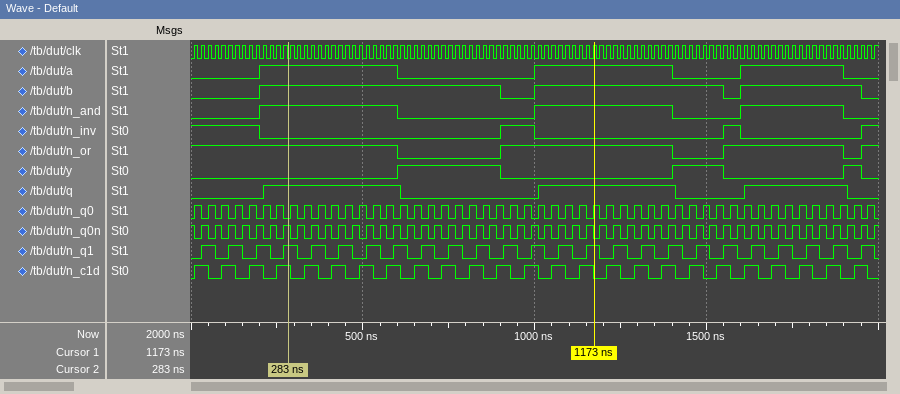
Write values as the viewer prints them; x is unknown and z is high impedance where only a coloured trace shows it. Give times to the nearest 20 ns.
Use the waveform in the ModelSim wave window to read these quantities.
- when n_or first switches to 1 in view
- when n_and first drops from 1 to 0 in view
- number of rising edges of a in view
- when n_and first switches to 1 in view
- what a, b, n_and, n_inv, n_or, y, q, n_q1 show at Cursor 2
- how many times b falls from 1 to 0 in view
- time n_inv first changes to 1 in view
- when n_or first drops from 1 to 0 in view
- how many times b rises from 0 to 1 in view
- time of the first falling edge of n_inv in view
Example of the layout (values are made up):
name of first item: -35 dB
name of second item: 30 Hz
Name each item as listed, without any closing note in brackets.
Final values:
when n_or first switches to 1 in view: 900 ns
when n_and first drops from 1 to 0 in view: 600 ns
number of rising edges of a in view: 3
when n_and first switches to 1 in view: 200 ns
what a, b, n_and, n_inv, n_or, y, q, n_q1 show at Cursor 2: a=1, b=1, n_and=1, n_inv=0, n_or=1, y=0, q=1, n_q1=1
how many times b falls from 1 to 0 in view: 3
time n_inv first changes to 1 in view: 900 ns
when n_or first drops from 1 to 0 in view: 600 ns
how many times b rises from 0 to 1 in view: 3
time of the first falling edge of n_inv in view: 200 ns
